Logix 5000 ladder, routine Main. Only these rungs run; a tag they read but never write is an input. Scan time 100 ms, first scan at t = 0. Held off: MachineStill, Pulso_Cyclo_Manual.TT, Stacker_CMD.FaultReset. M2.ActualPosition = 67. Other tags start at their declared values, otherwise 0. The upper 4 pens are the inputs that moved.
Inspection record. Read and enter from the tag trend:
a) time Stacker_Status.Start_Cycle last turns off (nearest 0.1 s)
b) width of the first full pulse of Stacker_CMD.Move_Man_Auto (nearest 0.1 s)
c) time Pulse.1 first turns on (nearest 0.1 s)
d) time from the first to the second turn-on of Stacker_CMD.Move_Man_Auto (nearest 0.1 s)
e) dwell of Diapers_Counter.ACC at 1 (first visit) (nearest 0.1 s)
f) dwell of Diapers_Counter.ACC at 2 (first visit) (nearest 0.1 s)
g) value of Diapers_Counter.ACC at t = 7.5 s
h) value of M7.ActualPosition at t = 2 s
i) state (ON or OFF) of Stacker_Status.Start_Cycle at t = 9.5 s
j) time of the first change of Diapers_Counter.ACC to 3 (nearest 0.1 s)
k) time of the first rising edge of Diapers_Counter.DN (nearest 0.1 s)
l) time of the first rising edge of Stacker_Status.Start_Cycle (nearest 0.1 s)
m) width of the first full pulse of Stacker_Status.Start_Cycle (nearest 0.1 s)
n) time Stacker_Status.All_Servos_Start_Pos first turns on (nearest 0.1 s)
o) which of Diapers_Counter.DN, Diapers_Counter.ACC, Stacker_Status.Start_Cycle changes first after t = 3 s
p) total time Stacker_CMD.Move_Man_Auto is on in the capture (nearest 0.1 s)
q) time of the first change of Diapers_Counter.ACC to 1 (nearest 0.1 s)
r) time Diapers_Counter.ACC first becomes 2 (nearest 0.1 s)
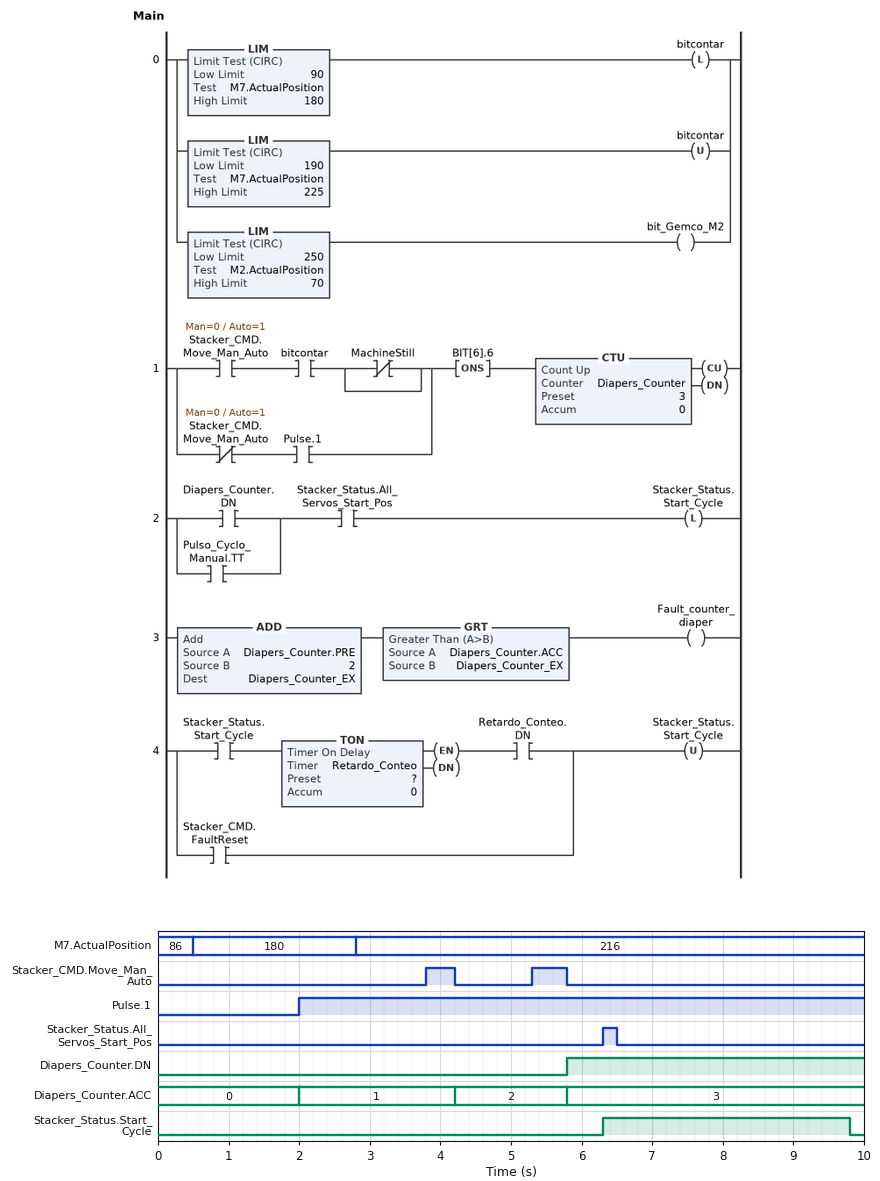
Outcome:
9.8 s
0.4 s
2.0 s
1.5 s
2.2 s
1.6 s
3
180
ON
5.8 s
5.8 s
6.3 s
3.5 s
6.3 s
Diapers_Counter.ACC
0.9 s
2.0 s
4.2 s
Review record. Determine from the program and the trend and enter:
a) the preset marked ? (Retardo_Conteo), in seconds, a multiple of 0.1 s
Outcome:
3.5 s
